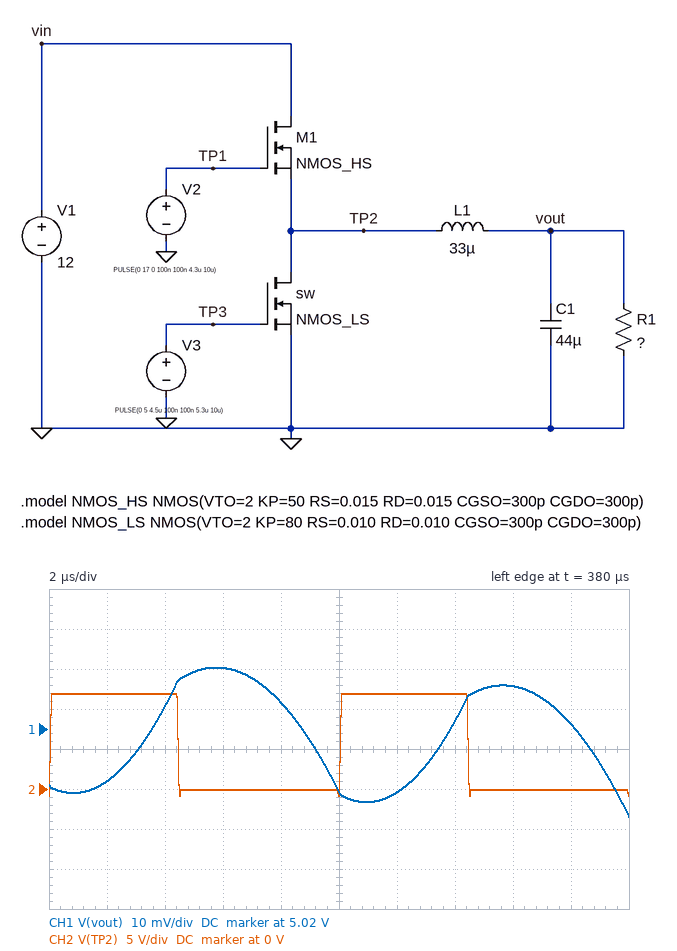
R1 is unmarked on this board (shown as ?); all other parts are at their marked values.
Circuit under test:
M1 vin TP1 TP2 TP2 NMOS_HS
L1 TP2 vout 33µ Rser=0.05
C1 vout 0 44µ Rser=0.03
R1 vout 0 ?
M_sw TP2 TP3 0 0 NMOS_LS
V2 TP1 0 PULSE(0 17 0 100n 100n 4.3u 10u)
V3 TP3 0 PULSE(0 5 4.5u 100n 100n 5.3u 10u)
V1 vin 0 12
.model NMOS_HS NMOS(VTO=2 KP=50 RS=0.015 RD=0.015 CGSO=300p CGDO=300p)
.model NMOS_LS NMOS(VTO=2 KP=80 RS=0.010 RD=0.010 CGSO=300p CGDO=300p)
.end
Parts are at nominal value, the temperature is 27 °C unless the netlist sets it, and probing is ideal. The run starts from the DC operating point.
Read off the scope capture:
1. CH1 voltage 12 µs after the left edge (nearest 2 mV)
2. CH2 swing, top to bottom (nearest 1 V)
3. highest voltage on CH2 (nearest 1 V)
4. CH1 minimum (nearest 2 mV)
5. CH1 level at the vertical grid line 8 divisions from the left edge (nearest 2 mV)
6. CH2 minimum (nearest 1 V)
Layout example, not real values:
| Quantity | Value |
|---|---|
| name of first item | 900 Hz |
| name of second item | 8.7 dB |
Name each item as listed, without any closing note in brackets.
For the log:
| Quantity | Value |
|---|---|
| CH1 voltage 12 µs after the left edge | 5.004 V |
| CH2 swing, top to bottom | 13 V |
| highest voltage on CH2 | 12 V |
| CH1 minimum | 4.998 V |
| CH1 level at the vertical grid line 8 divisions from the left edge | 5.030 V |
| CH2 minimum | -1 V |
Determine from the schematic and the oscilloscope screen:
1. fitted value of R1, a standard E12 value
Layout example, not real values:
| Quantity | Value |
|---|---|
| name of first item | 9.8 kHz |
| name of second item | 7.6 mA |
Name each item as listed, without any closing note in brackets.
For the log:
| Quantity | Value |
|---|---|
| fitted value of R1, a standard E12 value | 1.2 Ω |
